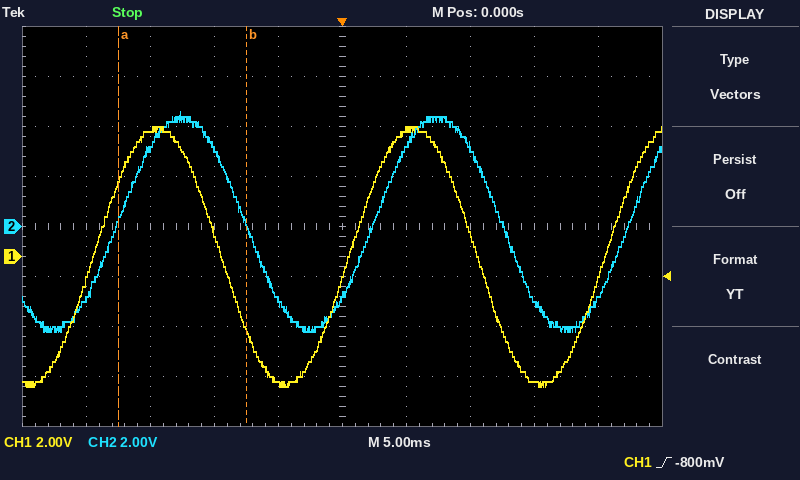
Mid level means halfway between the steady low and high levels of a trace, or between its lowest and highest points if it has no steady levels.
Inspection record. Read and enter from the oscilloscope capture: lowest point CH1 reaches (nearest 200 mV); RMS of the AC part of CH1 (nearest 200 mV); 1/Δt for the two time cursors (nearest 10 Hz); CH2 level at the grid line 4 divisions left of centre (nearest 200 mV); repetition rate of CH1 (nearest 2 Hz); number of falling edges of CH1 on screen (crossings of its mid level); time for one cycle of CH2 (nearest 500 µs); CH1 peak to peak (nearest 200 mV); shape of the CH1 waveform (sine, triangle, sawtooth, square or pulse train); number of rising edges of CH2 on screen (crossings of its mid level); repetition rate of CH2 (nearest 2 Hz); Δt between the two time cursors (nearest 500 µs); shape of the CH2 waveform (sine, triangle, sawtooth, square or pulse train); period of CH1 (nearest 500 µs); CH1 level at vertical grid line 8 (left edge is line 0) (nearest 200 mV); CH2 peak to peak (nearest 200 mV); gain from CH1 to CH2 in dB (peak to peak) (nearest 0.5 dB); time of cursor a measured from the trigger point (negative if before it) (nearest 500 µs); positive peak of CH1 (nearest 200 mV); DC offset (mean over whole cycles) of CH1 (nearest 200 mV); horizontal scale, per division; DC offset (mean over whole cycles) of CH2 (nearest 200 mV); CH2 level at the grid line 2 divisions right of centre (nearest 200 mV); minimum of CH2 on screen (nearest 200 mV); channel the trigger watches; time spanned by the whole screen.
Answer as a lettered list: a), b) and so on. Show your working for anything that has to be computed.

a) -5.2 V
b) 10.4 V / (2√2) ≈ 3.68 V, so 3.6 V to the nearest 200 mV
c) 1 / 10.0 ms ≈ 100 Hz
d) -2.8 V
e) 1 / 20.0 ms ≈ 50 Hz
f) 2
g) 20.0 ms
h) 5.2 V − (-5.2 V) = 10.4 V
i) sine
j) 3
k) 1 / 20.0 ms ≈ 50 Hz
l) 10.0 ms
m) sine
n) 20.0 ms
o) -5.0 V
p) 4.6 V − (-4.2 V) = 8.8 V
q) 20 log10(8.8 V / 10.4 V) ≈ -1.5 dB
r) -17.5 ms
s) 5.2 V
t) (5.2 V + (-5.2 V)) / 2 ≈ 0.0 V
u) 5 ms
v) (4.6 V + (-4.2 V)) / 2 ≈ 200 mV
w) 3.2 V
x) -4.2 V
y) CH1
z) 50 ms
